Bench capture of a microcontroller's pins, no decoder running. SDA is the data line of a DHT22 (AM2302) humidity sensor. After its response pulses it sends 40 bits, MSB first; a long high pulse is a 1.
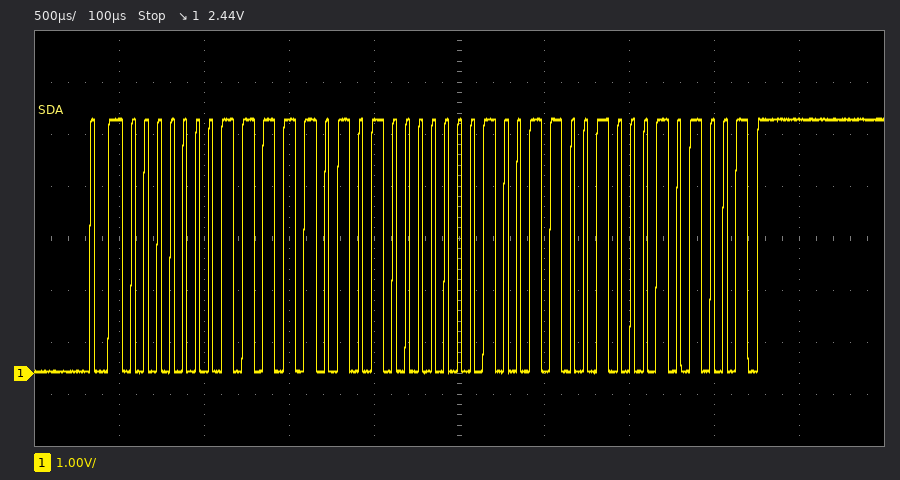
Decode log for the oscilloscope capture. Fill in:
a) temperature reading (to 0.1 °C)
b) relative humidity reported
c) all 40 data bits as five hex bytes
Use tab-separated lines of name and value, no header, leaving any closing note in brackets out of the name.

temperature reading	30.6 °C
relative humidity reported	50.1 %
all 40 data bits as five hex bytes	01 F5 01 32 29
